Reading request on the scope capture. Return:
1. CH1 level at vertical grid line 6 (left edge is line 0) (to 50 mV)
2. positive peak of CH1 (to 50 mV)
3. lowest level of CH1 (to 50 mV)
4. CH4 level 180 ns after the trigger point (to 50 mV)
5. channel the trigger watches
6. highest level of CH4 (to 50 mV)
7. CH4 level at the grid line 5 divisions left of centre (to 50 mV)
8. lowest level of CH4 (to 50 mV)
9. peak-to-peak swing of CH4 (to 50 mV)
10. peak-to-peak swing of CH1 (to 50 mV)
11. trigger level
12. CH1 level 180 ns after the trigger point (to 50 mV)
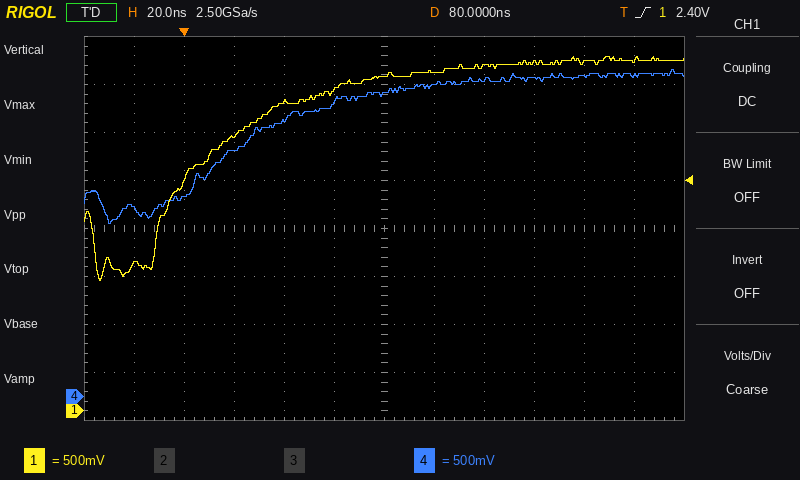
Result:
3.50 V
3.70 V
1.35 V
3.35 V
CH1
3.40 V
1.95 V
1.80 V
1.60 V
2.35 V
2.40 V
3.65 V
